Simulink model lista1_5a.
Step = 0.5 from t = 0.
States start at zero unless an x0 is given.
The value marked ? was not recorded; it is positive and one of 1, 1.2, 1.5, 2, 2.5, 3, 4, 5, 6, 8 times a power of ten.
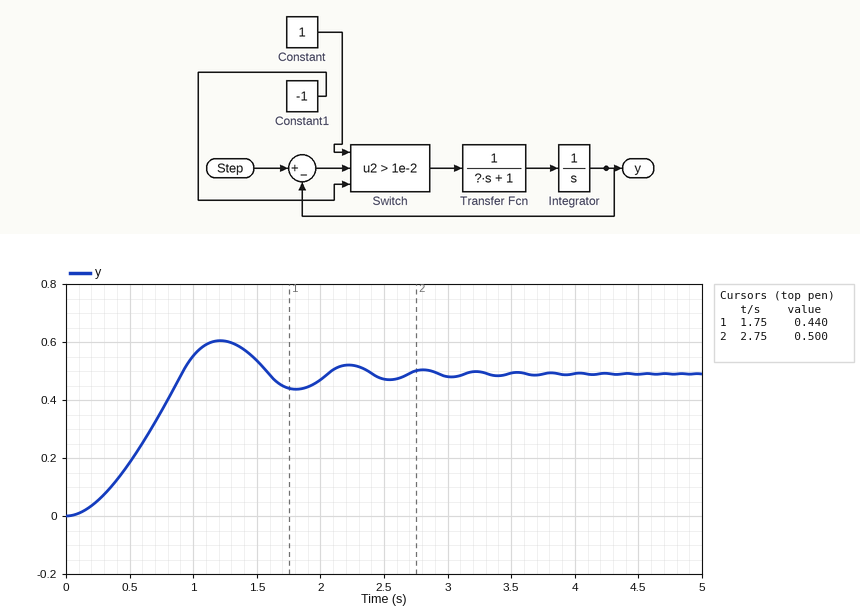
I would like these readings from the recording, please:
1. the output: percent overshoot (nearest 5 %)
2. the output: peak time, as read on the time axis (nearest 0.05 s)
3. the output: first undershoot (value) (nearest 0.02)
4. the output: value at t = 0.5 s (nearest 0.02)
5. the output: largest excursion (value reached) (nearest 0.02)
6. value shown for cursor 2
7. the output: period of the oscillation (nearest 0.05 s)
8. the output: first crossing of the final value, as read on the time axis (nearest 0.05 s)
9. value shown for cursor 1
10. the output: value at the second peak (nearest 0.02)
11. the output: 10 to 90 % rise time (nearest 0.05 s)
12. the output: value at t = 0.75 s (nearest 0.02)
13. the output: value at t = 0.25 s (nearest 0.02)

25 %
1.20 s
0.44
0.18
0.60
0.500
1.00 s
0.90 s
0.440
0.52
0.60 s
0.36
0.06
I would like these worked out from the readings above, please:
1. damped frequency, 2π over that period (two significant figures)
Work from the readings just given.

6.3 rad/s
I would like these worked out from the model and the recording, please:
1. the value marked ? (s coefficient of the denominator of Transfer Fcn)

0.5
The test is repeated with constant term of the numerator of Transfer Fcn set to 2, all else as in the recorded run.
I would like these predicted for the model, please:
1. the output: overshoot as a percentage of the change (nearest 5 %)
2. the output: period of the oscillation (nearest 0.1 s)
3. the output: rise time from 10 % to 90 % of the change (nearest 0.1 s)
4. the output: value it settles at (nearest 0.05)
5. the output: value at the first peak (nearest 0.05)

35 %
0.9 s
0.4 s
0.50
0.65
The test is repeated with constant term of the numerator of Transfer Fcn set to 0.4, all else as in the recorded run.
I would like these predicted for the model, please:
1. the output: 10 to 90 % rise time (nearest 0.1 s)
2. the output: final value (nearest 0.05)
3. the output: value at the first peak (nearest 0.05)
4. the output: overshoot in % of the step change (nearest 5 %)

1.2 s
0.50
0.55
10 %
